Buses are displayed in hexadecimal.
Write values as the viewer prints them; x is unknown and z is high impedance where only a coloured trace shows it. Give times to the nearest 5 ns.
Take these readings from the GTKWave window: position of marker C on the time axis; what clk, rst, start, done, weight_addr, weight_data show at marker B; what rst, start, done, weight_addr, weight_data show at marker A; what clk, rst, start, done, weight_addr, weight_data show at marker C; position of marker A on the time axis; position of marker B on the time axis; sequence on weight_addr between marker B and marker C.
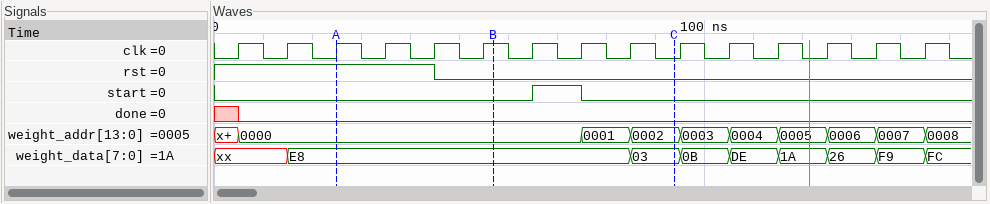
95 ns
clk=1, rst=0, start=0, done=0, weight_addr=0000, weight_data=E8
rst=1, start=0, done=0, weight_addr=0000, weight_data=E8
clk=0, rst=0, start=0, done=0, weight_addr=0002, weight_data=03
25 ns
55 ns
0000, 0001, 0002
